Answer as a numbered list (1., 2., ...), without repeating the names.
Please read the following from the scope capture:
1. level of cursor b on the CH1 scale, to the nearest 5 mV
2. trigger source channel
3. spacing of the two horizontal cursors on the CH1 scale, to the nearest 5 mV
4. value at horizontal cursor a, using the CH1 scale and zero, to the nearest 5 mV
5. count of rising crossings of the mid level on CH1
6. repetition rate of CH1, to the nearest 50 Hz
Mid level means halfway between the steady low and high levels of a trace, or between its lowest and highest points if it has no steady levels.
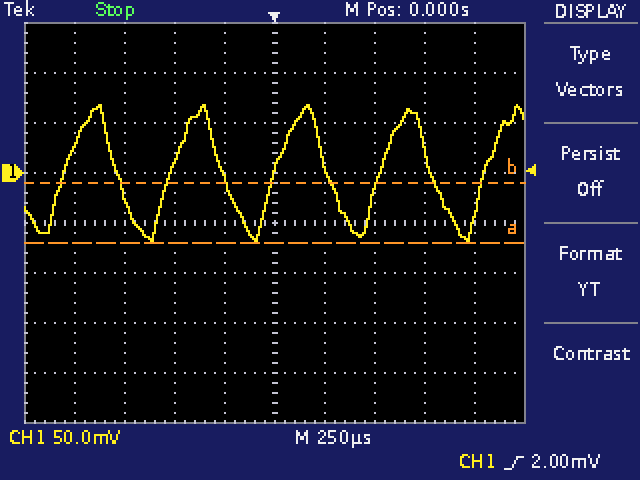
1. -10 mV
2. CH1
3. 60 mV
4. -70 mV
5. 5
6. 1.90 kHz
